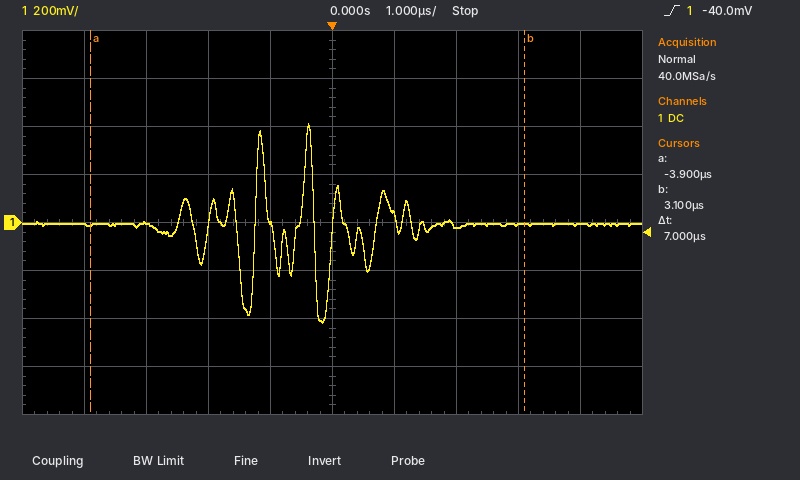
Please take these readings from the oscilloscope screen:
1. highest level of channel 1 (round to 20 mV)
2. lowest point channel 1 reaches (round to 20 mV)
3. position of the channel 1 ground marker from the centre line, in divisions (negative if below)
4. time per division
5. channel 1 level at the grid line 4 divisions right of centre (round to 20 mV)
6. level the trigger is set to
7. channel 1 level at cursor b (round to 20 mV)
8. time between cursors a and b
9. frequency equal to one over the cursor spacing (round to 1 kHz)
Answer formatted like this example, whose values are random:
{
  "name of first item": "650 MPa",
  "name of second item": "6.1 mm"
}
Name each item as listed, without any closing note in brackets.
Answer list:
{
  "highest level of channel 1": "420 mV",
  "lowest point channel 1 reaches": "-420 mV",
  "position of the channel 1 ground marker from the centre line, in divisions": "0.0 div",
  "time per division": "1 µs",
  "channel 1 level at the grid line 4 divisions right of centre": "0 mV",
  "level the trigger is set to": "-40.0 mV",
  "channel 1 level at cursor b": "0 mV",
  "time between cursors a and b": "7 µs",
  "frequency equal to one over the cursor spacing": "143 kHz"
}
